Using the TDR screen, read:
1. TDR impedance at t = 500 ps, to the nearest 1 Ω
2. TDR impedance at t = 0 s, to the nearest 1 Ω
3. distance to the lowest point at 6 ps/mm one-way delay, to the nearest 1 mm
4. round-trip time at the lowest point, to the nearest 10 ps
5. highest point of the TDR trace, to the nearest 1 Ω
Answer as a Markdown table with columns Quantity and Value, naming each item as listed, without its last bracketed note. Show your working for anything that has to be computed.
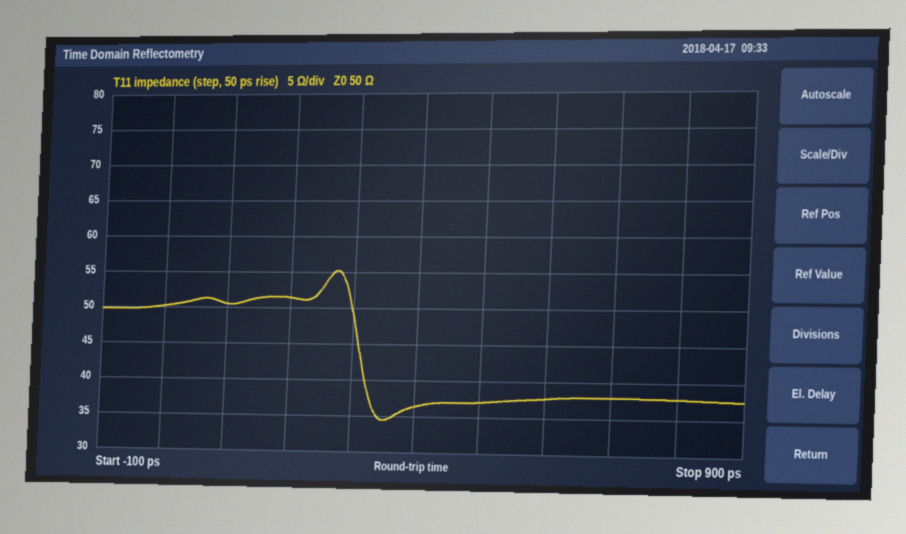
| Quantity | Value |
|---|---|
| TDR impedance at t = 500 ps, to the nearest 1 Ω | 37 Ω |
| TDR impedance at t = 0 s, to the nearest 1 Ω | 50 Ω |
| distance to the lowest point at 6 ps/mm one-way delay, to the nearest 1 mm | 350 ps / 2 / 6 ps/mm ≈ 29 mm |
| round-trip time at the lowest point, to the nearest 10 ps | 350 ps |
| highest point of the TDR trace, to the nearest 1 Ω | 55 Ω |
